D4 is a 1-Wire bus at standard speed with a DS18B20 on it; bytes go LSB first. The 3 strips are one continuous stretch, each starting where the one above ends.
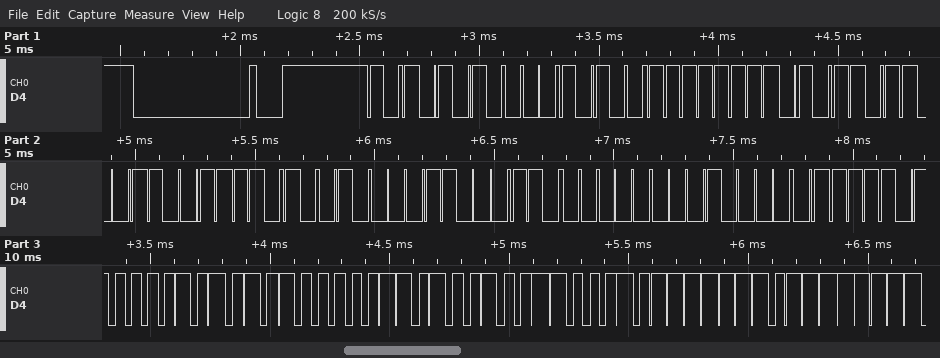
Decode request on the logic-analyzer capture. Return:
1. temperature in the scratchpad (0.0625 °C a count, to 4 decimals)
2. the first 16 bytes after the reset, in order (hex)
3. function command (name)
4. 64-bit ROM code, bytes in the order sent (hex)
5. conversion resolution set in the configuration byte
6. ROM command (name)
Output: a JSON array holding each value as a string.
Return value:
["85.0000 °C", "55 28 FF DA CC 4B 18 03 08 BE 50 05 4B 46 7F FF", "Read Scratchpad", "28 FF DA CC 4B 18 03 08", "12 bits", "Match ROM"]
